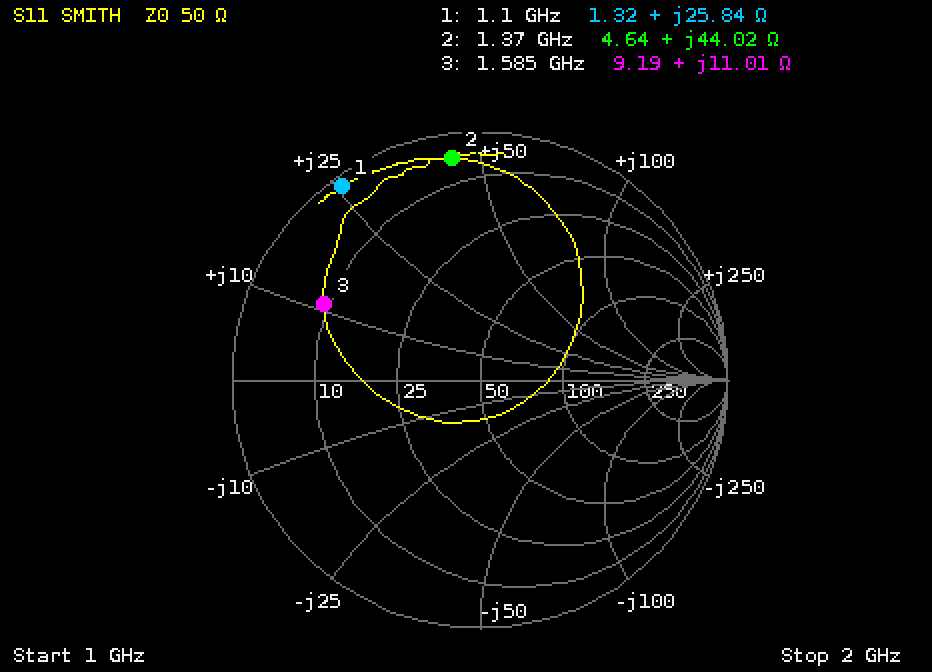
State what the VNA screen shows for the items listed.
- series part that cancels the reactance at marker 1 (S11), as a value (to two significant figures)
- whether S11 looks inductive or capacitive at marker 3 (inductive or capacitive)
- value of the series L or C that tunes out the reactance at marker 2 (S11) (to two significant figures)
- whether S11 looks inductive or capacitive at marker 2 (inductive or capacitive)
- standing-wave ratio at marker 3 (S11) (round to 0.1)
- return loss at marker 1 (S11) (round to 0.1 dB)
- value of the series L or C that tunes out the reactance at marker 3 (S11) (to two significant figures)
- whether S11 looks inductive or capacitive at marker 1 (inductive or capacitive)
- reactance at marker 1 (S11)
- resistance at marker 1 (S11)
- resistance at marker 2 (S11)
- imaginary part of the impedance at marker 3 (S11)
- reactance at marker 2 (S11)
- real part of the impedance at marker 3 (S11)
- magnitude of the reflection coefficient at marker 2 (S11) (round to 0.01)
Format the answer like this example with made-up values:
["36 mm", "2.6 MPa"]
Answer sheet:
["5.6 pF", "inductive", "2.6 pF", "inductive", "5.7", "0.4 dB", "9.1 pF", "inductive", "+25.84 Ω", "1.32 Ω", "4.64 Ω", "+11.01 Ω", "+44.02 Ω", "9.19 Ω", "0.90"]
